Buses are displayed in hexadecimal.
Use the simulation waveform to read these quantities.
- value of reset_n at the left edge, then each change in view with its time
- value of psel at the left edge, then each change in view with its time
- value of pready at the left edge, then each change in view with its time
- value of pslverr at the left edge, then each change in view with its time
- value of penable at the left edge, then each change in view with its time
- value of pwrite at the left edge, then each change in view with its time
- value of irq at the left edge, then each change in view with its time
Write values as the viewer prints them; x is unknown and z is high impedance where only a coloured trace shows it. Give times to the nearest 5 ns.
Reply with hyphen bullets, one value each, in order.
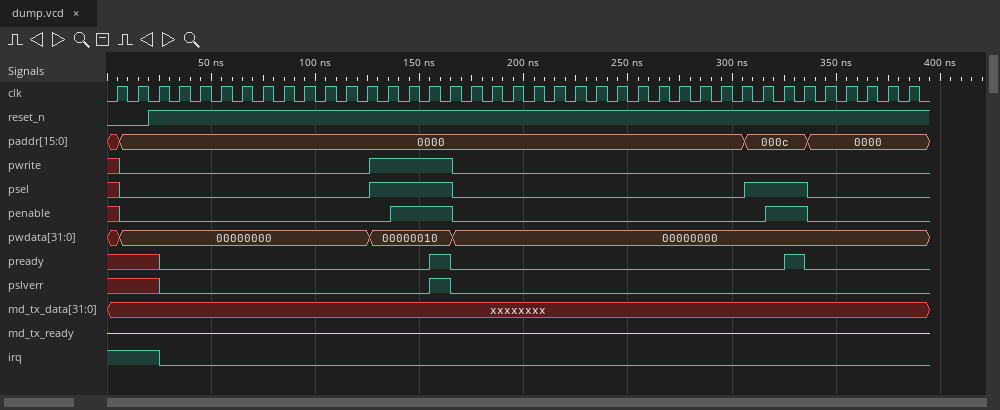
- 0, 1 at 20 ns
- x, 0 at 5 ns, 1 at 125 ns, 0 at 165 ns, 1 at 305 ns, 0 at 335 ns
- x, 0 at 25 ns, 1 at 155 ns, 0 at 165 ns, 1 at 325 ns, 0 at 335 ns
- x, 0 at 25 ns, 1 at 155 ns, 0 at 165 ns
- x, 0 at 5 ns, 1 at 135 ns, 0 at 165 ns, 1 at 315 ns, 0 at 335 ns
- x, 0 at 5 ns, 1 at 125 ns, 0 at 165 ns
- 1, 0 at 25 ns
